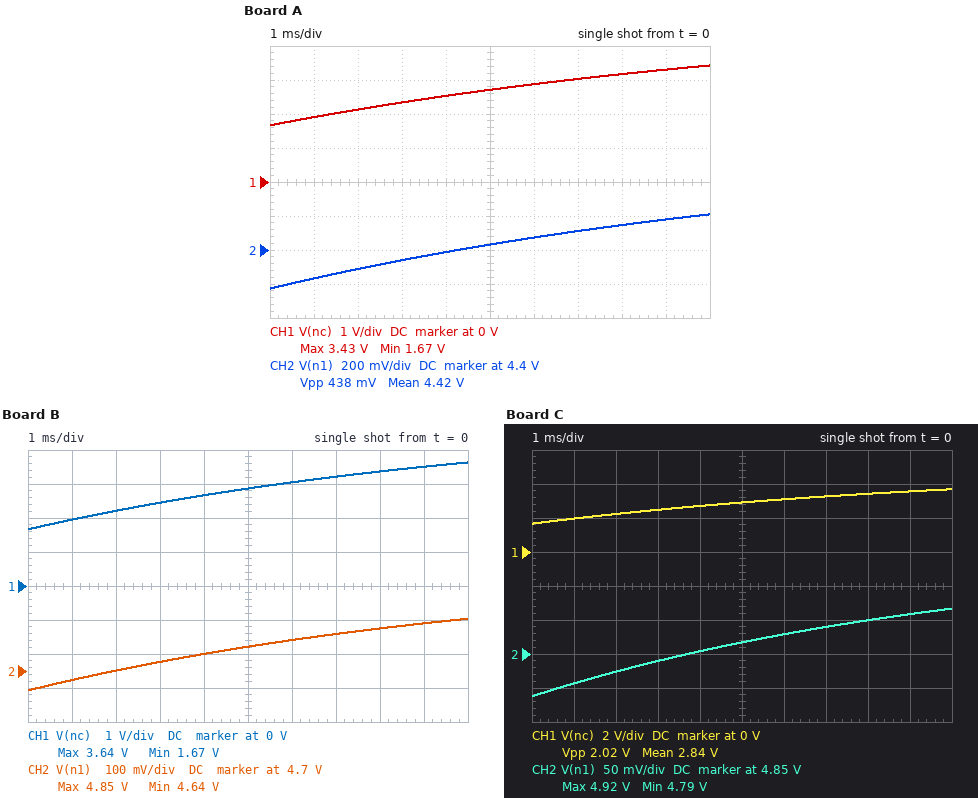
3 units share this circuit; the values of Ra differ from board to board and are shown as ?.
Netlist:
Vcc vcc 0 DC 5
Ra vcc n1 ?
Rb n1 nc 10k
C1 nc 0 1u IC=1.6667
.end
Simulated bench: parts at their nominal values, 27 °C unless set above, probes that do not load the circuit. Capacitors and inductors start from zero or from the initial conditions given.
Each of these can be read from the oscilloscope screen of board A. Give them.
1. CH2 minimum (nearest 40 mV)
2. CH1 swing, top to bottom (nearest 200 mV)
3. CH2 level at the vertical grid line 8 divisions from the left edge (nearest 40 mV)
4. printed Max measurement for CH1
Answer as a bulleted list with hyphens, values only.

- 4.16 V
- 1.8 V
- 4.56 V
- 3.43 V
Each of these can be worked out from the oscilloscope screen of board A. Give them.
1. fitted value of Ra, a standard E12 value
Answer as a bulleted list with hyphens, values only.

- 3.3 kΩ
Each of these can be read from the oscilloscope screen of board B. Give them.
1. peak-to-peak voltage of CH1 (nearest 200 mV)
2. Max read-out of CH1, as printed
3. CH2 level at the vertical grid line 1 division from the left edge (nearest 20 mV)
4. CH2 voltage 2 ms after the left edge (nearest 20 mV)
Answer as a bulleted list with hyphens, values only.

- 2.0 V
- 3.64 V
- 4.68 V
- 4.70 V
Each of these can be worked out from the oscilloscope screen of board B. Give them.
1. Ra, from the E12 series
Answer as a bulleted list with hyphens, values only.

- 1.2 kΩ
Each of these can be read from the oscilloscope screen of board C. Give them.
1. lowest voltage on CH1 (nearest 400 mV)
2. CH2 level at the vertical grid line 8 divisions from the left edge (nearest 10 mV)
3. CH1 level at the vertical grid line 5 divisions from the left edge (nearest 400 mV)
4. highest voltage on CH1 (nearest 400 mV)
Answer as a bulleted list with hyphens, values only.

- 1.6 V
- 4.90 V
- 2.8 V
- 3.6 V
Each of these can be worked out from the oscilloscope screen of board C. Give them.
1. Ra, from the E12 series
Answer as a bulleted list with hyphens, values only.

- 680 Ω
